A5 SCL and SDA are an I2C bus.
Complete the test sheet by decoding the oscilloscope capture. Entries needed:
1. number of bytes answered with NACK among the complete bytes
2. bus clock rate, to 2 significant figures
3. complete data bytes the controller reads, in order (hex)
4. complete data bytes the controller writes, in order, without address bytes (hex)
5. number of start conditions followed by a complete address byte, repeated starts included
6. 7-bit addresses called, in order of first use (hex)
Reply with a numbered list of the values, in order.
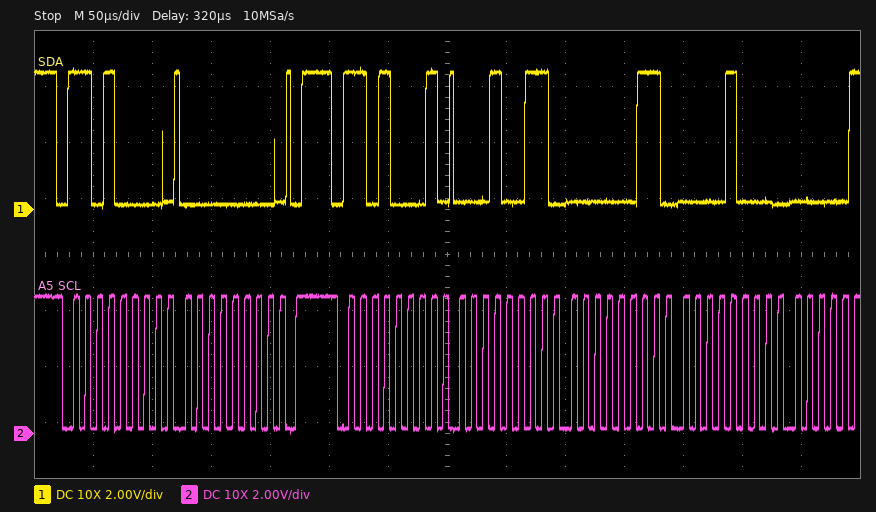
1. 0
2. 100 kHz
3. 13 03 08
4. 00
5. 2
6. 0x68
